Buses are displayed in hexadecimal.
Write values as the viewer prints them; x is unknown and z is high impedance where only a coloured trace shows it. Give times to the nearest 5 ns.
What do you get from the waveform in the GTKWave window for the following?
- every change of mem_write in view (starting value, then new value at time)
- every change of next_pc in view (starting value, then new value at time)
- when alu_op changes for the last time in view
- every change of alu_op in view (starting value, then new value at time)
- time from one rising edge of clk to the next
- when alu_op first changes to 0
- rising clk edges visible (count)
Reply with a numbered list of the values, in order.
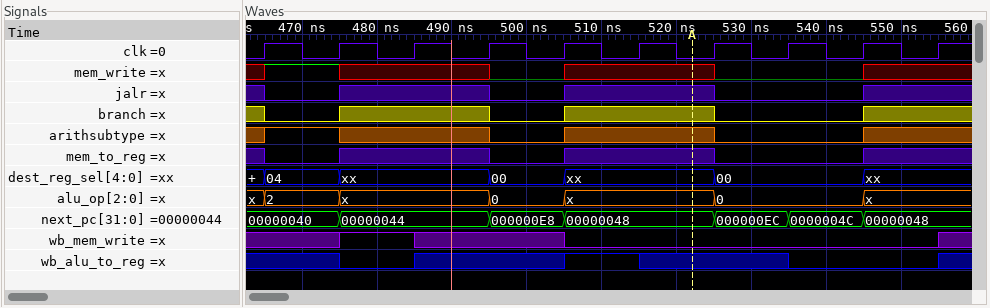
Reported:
1. x, 1 at 465 ns, x at 475 ns, 0 at 495 ns, x at 505 ns, 0 at 525 ns, x at 545 ns
2. 00000040, 00000044 at 475 ns, 000000E8 at 495 ns, 00000048 at 505 ns, 000000EC at 525 ns, 0000004C at 535 ns, 00000048 at 545 ns
3. 545 ns
4. x, 2 at 465 ns, x at 475 ns, 0 at 495 ns, x at 505 ns, 0 at 525 ns, x at 545 ns
5. 10 ns
6. 495 ns
7. 10
